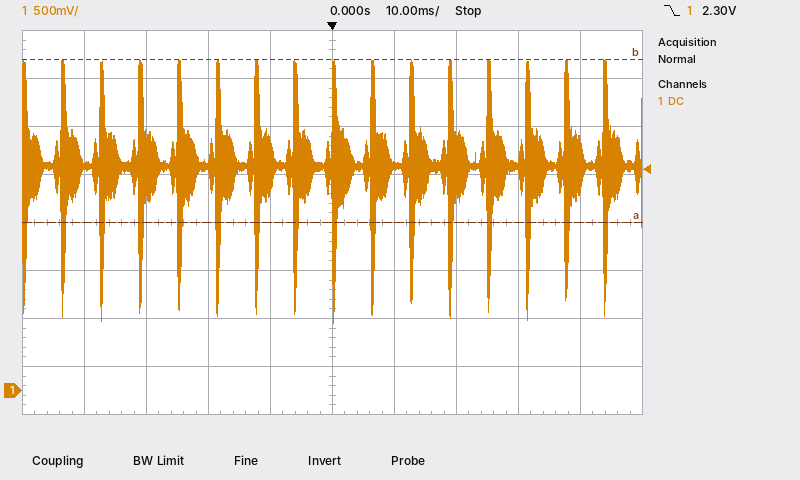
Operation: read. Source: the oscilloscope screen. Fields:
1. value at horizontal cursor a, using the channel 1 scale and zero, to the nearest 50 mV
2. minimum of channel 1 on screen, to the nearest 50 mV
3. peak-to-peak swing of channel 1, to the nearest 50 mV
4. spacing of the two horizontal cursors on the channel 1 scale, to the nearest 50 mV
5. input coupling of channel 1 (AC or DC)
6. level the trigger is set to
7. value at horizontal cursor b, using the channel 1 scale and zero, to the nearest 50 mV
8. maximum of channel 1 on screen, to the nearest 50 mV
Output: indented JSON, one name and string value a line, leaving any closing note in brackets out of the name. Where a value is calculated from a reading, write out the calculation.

{
  "value at horizontal cursor a, using the channel 1 scale and zero, to the nearest 50 mV": "1.75 V",
  "minimum of channel 1 on screen, to the nearest 50 mV": "700 mV",
  "peak-to-peak swing of channel 1, to the nearest 50 mV": "3.45 V − (700 mV) = 2.75 V",
  "spacing of the two horizontal cursors on the channel 1 scale, to the nearest 50 mV": "1.70 V",
  "input coupling of channel 1": "DC",
  "level the trigger is set to": "2.30 V",
  "value at horizontal cursor b, using the channel 1 scale and zero, to the nearest 50 mV": "3.45 V",
  "maximum of channel 1 on screen, to the nearest 50 mV": "3.45 V"
}
